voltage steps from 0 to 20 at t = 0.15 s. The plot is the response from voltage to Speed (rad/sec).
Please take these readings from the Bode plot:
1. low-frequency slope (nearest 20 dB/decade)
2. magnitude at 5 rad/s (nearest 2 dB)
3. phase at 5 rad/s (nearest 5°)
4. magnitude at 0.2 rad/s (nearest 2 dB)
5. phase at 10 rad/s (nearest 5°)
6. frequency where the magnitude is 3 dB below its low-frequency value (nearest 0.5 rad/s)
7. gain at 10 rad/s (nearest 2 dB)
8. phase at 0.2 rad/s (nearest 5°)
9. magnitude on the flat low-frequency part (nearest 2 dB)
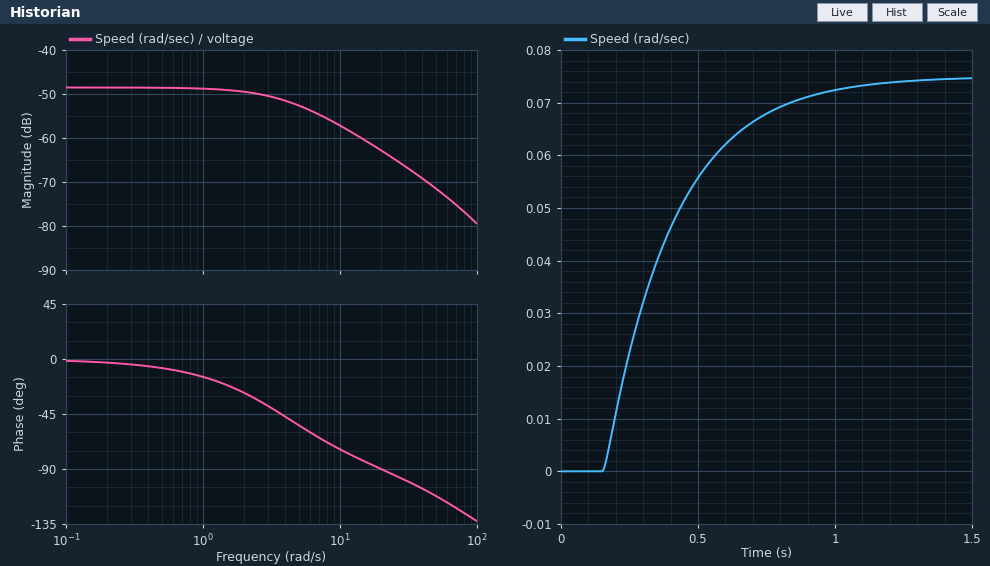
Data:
0 dB/decade
-52 dB
-55°
-48 dB
-75°
4.0 rad/s
-58 dB
-5°
-48 dB
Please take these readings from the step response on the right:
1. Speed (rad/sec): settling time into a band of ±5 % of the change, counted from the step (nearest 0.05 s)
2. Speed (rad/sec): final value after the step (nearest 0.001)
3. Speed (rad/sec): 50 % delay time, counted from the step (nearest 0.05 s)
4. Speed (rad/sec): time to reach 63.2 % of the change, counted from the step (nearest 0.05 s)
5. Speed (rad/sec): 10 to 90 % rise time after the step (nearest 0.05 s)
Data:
0.75 s
0.075
0.20 s
0.25 s
0.55 s
